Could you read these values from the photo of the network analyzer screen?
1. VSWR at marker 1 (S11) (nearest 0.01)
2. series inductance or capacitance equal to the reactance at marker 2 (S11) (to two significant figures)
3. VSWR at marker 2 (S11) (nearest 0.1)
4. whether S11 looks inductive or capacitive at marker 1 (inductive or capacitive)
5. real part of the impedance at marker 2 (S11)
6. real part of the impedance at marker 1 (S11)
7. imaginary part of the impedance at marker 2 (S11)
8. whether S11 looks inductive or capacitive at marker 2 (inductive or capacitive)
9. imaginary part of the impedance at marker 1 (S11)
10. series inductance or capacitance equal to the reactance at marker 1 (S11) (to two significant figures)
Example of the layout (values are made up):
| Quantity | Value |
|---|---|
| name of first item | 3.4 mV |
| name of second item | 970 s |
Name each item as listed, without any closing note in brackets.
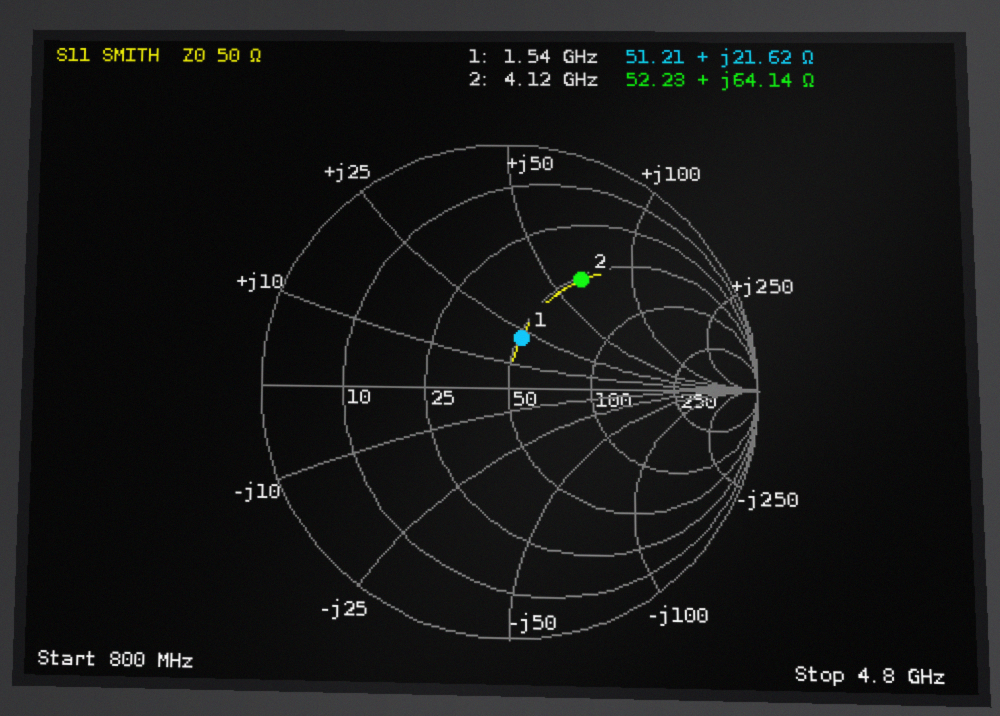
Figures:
| Quantity | Value |
|---|---|
| VSWR at marker 1 (S11) | 1.53 |
| series inductance or capacitance equal to the reactance at marker 2 (S11) | 2.5 nH |
| VSWR at marker 2 (S11) | 3.3 |
| whether S11 looks inductive or capacitive at marker 1 | inductive |
| real part of the impedance at marker 2 | 52.23 Ω |
| real part of the impedance at marker 1 | 51.21 Ω |
| imaginary part of the impedance at marker 2 | +64.14 Ω |
| whether S11 looks inductive or capacitive at marker 2 | inductive |
| imaginary part of the impedance at marker 1 | +21.62 Ω |
| series inductance or capacitance equal to the reactance at marker 1 (S11) | 2.2 nH |
